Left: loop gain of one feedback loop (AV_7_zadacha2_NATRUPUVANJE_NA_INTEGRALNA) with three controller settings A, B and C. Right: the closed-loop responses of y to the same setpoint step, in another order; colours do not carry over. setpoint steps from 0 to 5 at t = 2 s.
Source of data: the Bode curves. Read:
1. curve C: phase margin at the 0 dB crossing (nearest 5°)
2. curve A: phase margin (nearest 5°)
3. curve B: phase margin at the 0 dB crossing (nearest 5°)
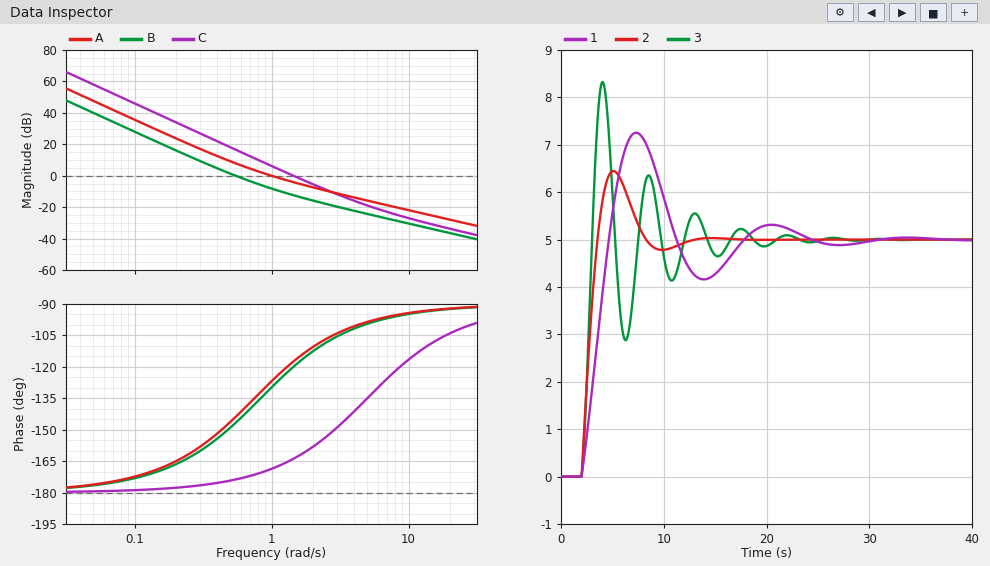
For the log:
15°
55°
35°
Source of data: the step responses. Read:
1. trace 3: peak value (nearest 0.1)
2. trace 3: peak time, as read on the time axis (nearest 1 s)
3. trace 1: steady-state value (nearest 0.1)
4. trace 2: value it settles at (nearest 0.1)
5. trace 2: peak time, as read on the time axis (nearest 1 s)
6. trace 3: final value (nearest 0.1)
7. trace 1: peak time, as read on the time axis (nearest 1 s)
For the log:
8.3
4 s
5.0
5.0
5 s
5.0
7 s
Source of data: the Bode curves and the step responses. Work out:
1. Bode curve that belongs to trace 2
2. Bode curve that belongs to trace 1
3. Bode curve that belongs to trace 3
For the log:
A
B
C
